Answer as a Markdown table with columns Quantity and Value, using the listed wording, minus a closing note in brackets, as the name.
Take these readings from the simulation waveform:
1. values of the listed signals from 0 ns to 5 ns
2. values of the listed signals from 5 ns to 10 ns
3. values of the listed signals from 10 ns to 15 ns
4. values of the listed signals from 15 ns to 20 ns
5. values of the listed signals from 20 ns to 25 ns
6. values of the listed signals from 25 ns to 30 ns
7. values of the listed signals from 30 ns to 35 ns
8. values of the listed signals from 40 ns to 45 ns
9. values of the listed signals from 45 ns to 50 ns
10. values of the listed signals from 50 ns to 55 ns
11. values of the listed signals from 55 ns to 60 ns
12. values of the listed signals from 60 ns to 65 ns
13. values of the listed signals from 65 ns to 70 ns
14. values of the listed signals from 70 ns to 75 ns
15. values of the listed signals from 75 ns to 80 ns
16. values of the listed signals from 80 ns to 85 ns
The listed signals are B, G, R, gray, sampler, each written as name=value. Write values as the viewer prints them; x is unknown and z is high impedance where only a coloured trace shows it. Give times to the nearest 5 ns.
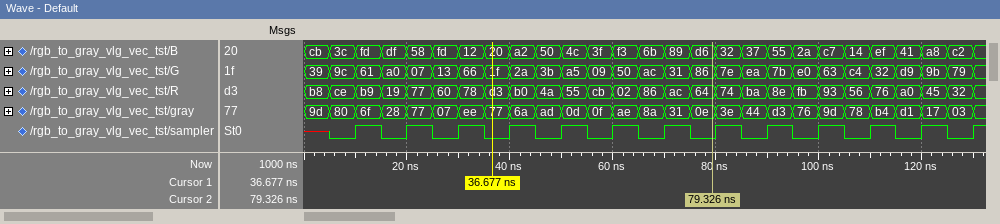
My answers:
| Quantity | Value |
|---|---|
| values of the listed signals from 0 ns to 5 ns | B=cb, G=39, R=b8, gray=9d, sampler=x |
| values of the listed signals from 5 ns to 10 ns | B=3c, G=9c, R=ce, gray=80, sampler=0 |
| values of the listed signals from 10 ns to 15 ns | B=fd, G=61, R=b9, gray=6f, sampler=1 |
| values of the listed signals from 15 ns to 20 ns | B=df, G=a0, R=19, gray=28, sampler=0 |
| values of the listed signals from 20 ns to 25 ns | B=58, G=07, R=77, gray=77, sampler=1 |
| values of the listed signals from 25 ns to 30 ns | B=fd, G=13, R=60, gray=07, sampler=0 |
| values of the listed signals from 30 ns to 35 ns | B=12, G=66, R=78, gray=ee, sampler=1 |
| values of the listed signals from 40 ns to 45 ns | B=a2, G=2a, R=b0, gray=6a, sampler=1 |
| values of the listed signals from 45 ns to 50 ns | B=50, G=3b, R=4a, gray=ad, sampler=0 |
| values of the listed signals from 50 ns to 55 ns | B=4c, G=a5, R=55, gray=0d, sampler=1 |
| values of the listed signals from 55 ns to 60 ns | B=3f, G=09, R=cb, gray=0f, sampler=0 |
| values of the listed signals from 60 ns to 65 ns | B=f3, G=50, R=02, gray=ae, sampler=1 |
| values of the listed signals from 65 ns to 70 ns | B=6b, G=ac, R=86, gray=8a, sampler=0 |
| values of the listed signals from 70 ns to 75 ns | B=89, G=31, R=ac, gray=31, sampler=1 |
| values of the listed signals from 75 ns to 80 ns | B=d6, G=86, R=64, gray=0e, sampler=0 |
| values of the listed signals from 80 ns to 85 ns | B=32, G=7e, R=74, gray=3e, sampler=1 |
